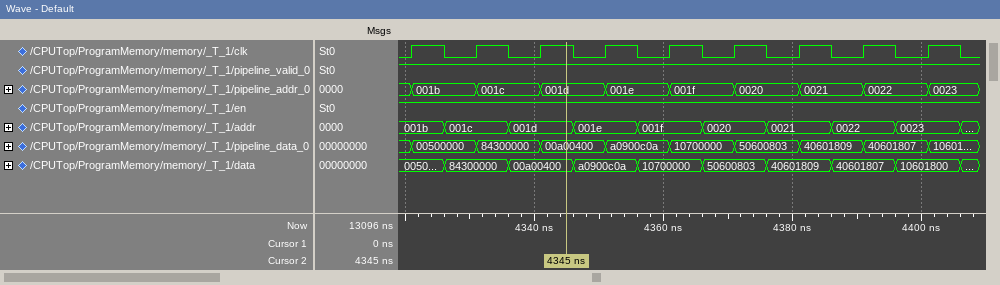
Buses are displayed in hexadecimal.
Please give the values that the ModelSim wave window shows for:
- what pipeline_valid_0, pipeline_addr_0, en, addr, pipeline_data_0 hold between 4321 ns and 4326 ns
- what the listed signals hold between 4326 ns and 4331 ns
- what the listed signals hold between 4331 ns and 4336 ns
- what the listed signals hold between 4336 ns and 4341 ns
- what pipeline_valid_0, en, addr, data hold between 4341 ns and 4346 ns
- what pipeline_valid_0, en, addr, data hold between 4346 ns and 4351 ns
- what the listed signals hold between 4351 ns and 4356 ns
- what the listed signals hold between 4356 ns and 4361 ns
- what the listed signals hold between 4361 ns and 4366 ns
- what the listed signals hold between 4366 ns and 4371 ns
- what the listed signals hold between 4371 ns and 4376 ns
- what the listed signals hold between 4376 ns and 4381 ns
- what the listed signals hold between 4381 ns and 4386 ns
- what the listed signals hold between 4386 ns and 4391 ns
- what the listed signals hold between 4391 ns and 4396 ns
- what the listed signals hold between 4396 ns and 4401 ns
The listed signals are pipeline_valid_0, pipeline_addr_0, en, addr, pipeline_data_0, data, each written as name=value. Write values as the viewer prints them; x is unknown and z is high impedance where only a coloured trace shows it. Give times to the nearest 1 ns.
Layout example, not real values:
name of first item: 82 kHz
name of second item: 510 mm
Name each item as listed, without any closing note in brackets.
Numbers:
what pipeline_valid_0, pipeline_addr_0, en, addr, pipeline_data_0 hold between 4321 ns and 4326 ns: pipeline_valid_0=1, pipeline_addr_0=001b, en=1, addr=001b, pipeline_data_0=00500000
what the listed signals hold between 4326 ns and 4331 ns: pipeline_valid_0=1, pipeline_addr_0=001b, en=1, addr=001c, pipeline_data_0=00500000, data=84300000
what the listed signals hold between 4331 ns and 4336 ns: pipeline_valid_0=1, pipeline_addr_0=001c, en=1, addr=001c, pipeline_data_0=84300000, data=84300000
what the listed signals hold between 4336 ns and 4341 ns: pipeline_valid_0=1, pipeline_addr_0=001c, en=1, addr=001d, pipeline_data_0=84300000, data=00a00400
what pipeline_valid_0, en, addr, data hold between 4341 ns and 4346 ns: pipeline_valid_0=1, en=1, addr=001d, data=00a00400
what pipeline_valid_0, en, addr, data hold between 4346 ns and 4351 ns: pipeline_valid_0=1, en=1, addr=001e, data=a0900c0a
what the listed signals hold between 4351 ns and 4356 ns: pipeline_valid_0=1, pipeline_addr_0=001e, en=1, addr=001e, pipeline_data_0=a0900c0a, data=a0900c0a
what the listed signals hold between 4356 ns and 4361 ns: pipeline_valid_0=1, pipeline_addr_0=001e, en=1, addr=001f, pipeline_data_0=a0900c0a, data=10700000
what the listed signals hold between 4361 ns and 4366 ns: pipeline_valid_0=1, pipeline_addr_0=001f, en=1, addr=001f, pipeline_data_0=10700000, data=10700000
what the listed signals hold between 4366 ns and 4371 ns: pipeline_valid_0=1, pipeline_addr_0=001f, en=1, addr=0020, pipeline_data_0=10700000, data=50600803
what the listed signals hold between 4371 ns and 4376 ns: pipeline_valid_0=1, pipeline_addr_0=0020, en=1, addr=0020, pipeline_data_0=50600803, data=50600803
what the listed signals hold between 4376 ns and 4381 ns: pipeline_valid_0=1, pipeline_addr_0=0020, en=1, addr=0021, pipeline_data_0=50600803, data=40601809
what the listed signals hold between 4381 ns and 4386 ns: pipeline_valid_0=1, pipeline_addr_0=0021, en=1, addr=0021, pipeline_data_0=40601809, data=40601809
what the listed signals hold between 4386 ns and 4391 ns: pipeline_valid_0=1, pipeline_addr_0=0021, en=1, addr=0022, pipeline_data_0=40601809, data=40601807
what the listed signals hold between 4391 ns and 4396 ns: pipeline_valid_0=1, pipeline_addr_0=0022, en=1, addr=0022, pipeline_data_0=40601807, data=40601807
what the listed signals hold between 4396 ns and 4401 ns: pipeline_valid_0=1, pipeline_addr_0=0022, en=1, addr=0023, pipeline_data_0=40601807, data=10601800
